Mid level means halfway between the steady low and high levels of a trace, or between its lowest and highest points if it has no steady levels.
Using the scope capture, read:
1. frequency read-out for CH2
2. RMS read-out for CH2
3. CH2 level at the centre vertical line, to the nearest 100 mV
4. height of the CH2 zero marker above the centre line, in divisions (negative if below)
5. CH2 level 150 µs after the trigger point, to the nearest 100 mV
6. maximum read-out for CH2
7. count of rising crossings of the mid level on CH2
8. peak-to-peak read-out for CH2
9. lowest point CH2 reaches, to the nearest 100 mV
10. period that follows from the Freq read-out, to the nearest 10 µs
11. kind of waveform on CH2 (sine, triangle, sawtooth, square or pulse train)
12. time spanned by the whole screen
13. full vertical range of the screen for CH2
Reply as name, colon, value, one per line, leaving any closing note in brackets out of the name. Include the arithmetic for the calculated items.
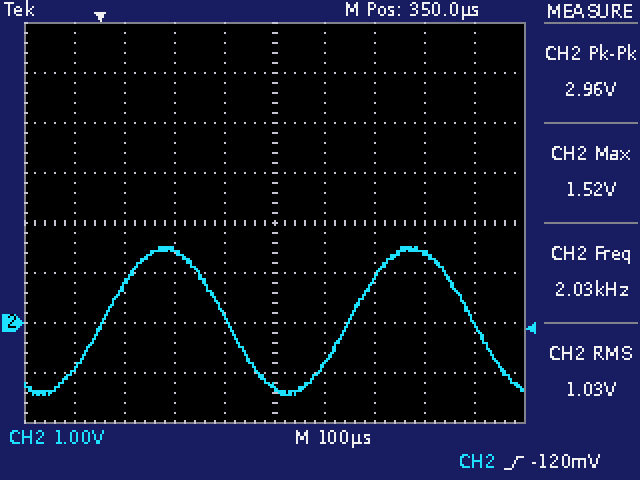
frequency read-out for CH2: 2.03 kHz
RMS read-out for CH2: 1.03 V
CH2 level at the centre vertical line, to the nearest 100 mV: -1.3 V
height of the CH2 zero marker above the centre line, in divisions: -2.0 div
CH2 level 150 µs after the trigger point, to the nearest 100 mV: 1.4 V
maximum read-out for CH2: 1.52 V
count of rising crossings of the mid level on CH2: 2
peak-to-peak read-out for CH2: 2.96 V
lowest point CH2 reaches, to the nearest 100 mV: -1.4 V
period that follows from the Freq read-out, to the nearest 10 µs: 1 / 2.03 kHz ≈ 493 µs, so 490 µs to the nearest 10 µs
kind of waveform on CH2: sine
time spanned by the whole screen: 1 ms
full vertical range of the screen for CH2: 8 V
